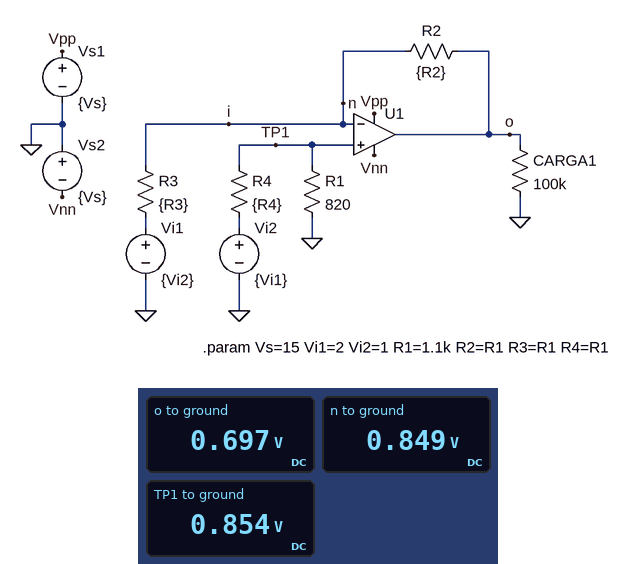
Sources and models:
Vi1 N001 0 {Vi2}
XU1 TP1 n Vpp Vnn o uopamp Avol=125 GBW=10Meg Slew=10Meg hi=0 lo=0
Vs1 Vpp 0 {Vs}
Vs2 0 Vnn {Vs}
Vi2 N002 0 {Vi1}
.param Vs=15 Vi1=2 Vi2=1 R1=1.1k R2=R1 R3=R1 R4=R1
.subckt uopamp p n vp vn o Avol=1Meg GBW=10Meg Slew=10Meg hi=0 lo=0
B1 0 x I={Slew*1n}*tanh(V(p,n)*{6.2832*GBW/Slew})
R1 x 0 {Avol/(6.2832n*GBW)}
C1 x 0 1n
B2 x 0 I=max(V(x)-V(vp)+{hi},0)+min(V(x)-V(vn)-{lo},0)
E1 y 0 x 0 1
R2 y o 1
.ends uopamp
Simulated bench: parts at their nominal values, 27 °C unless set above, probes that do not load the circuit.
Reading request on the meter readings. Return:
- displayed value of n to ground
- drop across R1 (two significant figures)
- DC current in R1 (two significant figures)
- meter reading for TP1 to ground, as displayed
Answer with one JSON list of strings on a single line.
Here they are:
["0.849 V", "850 mV", "1.0 mA", "0.854 V"]
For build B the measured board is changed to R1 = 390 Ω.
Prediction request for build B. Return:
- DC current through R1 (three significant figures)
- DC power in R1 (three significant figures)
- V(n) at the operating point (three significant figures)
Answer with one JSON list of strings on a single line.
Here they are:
["1.34 mA", "703 µW", "523 mV"]
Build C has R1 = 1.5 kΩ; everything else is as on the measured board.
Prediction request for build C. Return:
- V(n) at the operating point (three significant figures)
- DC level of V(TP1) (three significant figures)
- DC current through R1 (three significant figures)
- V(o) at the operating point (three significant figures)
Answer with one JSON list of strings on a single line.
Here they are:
["1.14 V", "1.15 V", "769 µA", "1.29 V"]
